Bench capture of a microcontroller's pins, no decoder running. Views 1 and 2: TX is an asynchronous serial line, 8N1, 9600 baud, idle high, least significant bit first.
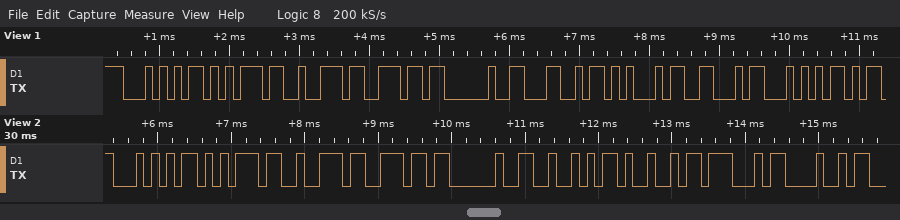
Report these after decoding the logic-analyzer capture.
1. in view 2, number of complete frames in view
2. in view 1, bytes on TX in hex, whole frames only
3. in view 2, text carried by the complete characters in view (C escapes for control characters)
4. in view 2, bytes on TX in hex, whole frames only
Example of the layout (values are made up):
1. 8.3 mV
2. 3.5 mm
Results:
1. 9
2. 54 75 72 6E 20 4C 45 46 54
3. "Turn RIGH"
4. 54 75 72 6E 20 52 49 47 48
